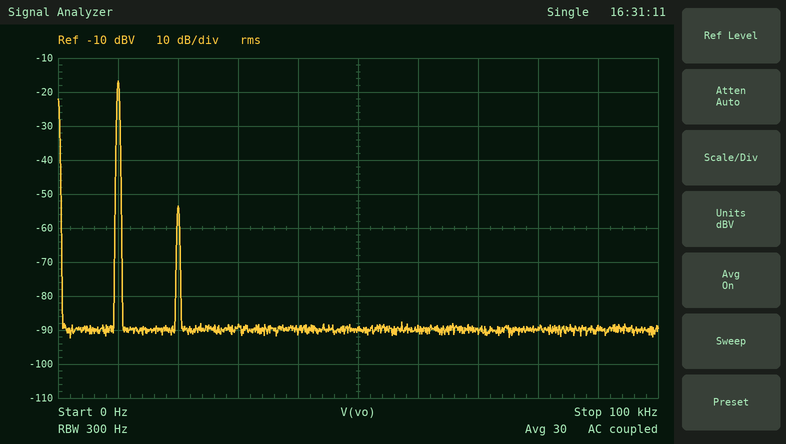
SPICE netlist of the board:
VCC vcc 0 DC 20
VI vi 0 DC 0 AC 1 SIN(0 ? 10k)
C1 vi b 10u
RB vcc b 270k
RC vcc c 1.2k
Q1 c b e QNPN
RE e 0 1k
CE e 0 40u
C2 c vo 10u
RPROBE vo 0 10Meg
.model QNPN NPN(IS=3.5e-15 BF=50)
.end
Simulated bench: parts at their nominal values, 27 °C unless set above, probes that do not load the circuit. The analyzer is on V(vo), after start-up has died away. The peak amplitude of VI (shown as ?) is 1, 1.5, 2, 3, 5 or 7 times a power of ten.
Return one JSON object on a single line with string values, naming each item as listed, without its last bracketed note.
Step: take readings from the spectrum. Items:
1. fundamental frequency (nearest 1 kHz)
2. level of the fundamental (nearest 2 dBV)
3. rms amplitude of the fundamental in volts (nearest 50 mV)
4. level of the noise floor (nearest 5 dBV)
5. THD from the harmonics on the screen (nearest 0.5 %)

{"fundamental frequency": "10 kHz", "level of the fundamental": "-16 dBV", "rms amplitude of the fundamental in volts": "150 mV", "level of the noise floor": "-90 dBV", "THD from the harmonics on the screen": "1.5 %"}
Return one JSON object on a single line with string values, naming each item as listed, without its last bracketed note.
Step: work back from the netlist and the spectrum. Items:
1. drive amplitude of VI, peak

{"drive amplitude of VI, peak": "1.5 mV"}
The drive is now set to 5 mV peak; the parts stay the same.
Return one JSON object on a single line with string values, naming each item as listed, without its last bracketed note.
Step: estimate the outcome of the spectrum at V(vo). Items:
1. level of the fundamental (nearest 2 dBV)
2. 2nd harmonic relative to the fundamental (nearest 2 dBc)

{"level of the fundamental": "-6 dBV", "2nd harmonic relative to the fundamental": "-26 dBc"}
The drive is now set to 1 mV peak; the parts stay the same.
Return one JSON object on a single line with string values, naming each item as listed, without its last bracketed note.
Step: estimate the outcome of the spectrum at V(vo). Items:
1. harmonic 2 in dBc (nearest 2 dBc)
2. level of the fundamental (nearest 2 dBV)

{"harmonic 2 in dBc": "-40 dBc", "level of the fundamental": "-20 dBV"}
